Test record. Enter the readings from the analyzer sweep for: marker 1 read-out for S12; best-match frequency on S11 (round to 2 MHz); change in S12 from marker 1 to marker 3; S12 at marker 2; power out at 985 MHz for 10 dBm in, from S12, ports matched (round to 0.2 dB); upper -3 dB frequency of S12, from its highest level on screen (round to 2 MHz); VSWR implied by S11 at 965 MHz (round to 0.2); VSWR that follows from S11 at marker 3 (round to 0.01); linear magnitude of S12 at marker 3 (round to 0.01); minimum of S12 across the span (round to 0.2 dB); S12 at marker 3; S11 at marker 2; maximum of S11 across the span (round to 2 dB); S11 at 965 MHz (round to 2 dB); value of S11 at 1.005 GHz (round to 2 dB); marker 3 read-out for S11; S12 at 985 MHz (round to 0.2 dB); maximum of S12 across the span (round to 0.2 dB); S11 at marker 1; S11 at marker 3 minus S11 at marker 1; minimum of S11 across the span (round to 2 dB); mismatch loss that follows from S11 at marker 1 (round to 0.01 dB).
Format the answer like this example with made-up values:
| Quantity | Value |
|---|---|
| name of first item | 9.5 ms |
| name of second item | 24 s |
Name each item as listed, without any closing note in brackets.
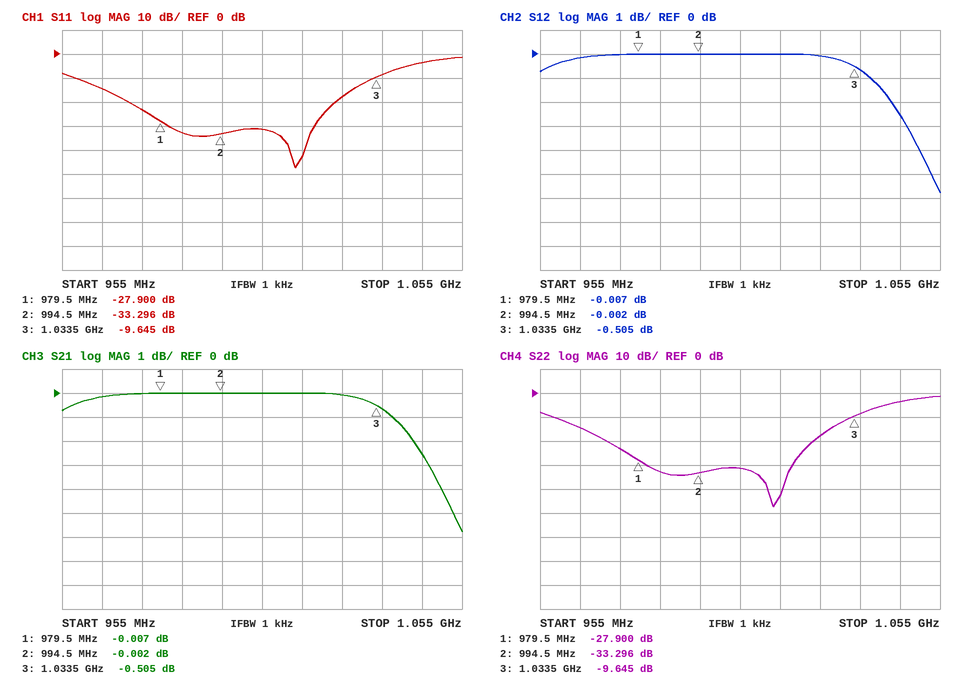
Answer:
| Quantity | Value |
|---|---|
| marker 1 read-out for S12 | -0.007 dB |
| best-match frequency on S11 | 1.014 GHz |
| change in S12 from marker 1 to marker 3 | -0.498 dB |
| S12 at marker 2 | -0.002 dB |
| power out at 985 MHz for 10 dBm in, from S12, ports matched | 10.0 dBm |
| upper -3 dB frequency of S12, from its highest level on screen | 1.046 GHz |
| VSWR implied by S11 at 965 MHz | 1.4 |
| VSWR that follows from S11 at marker 3 | 1.98 |
| linear magnitude of S12 at marker 3 | 0.94 |
| minimum of S12 across the span | -5.8 dB |
| S12 at marker 3 | -0.505 dB |
| S11 at marker 2 | -33.296 dB |
| maximum of S11 across the span | -2 dB |
| S11 at 965 MHz | -14 dB |
| value of S11 at 1.005 GHz | -32 dB |
| marker 3 read-out for S11 | -9.645 dB |
| S12 at 985 MHz | 0.0 dB |
| maximum of S12 across the span | 0.0 dB |
| S11 at marker 1 | -27.900 dB |
| S11 at marker 3 minus S11 at marker 1 | 18.255 dB |
| minimum of S11 across the span | -48 dB |
| mismatch loss that follows from S11 at marker 1 | 0.01 dB |
